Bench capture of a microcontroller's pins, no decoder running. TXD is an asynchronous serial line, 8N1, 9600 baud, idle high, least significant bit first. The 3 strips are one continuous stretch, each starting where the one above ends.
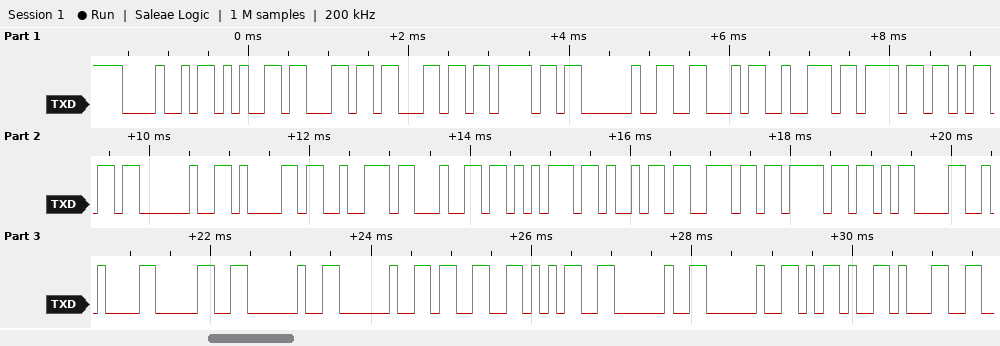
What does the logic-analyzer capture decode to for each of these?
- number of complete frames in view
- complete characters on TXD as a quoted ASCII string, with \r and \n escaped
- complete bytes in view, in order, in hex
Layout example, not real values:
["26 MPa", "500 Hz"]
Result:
["29", "\"Hello From arduino\\r\\n0  35  -1\"", "48 65 6C 6C 6F 20 46 72 6F 6D 20 61 72 64 75 69 6E 6F 0D 0A 30 20 20 33 35 20 20 2D 31"]
